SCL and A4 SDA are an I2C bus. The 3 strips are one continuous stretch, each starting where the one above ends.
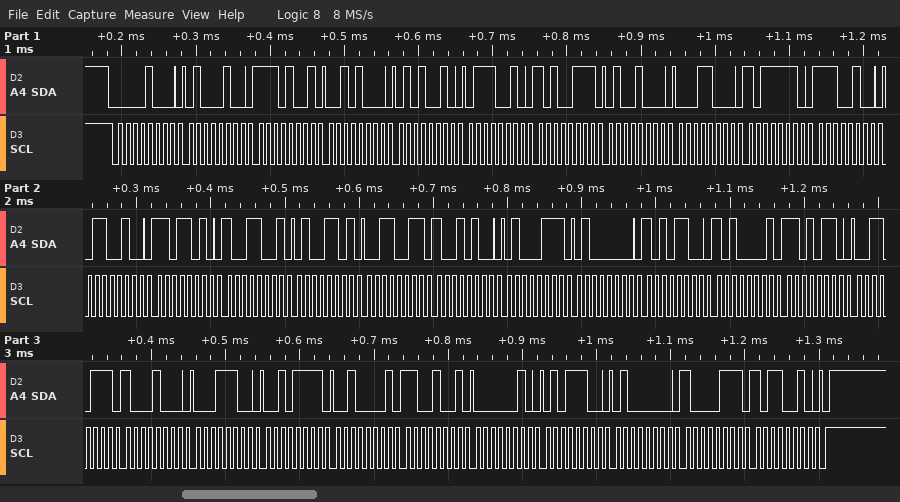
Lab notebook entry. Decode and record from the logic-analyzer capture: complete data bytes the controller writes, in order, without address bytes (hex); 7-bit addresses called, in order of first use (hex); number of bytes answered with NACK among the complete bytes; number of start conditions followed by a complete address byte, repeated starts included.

44 E9 28 52 72 A7 48 18 BE E4 64 DA 99 4D 33 94 47 40 AC A1 D6 37 88 1C 2F 21 C9 02 5C 40 87 B2
0x04
0
1
